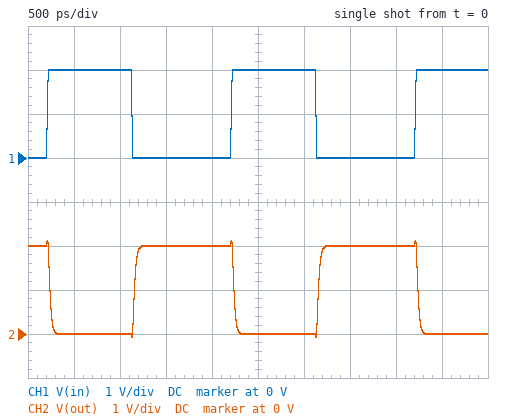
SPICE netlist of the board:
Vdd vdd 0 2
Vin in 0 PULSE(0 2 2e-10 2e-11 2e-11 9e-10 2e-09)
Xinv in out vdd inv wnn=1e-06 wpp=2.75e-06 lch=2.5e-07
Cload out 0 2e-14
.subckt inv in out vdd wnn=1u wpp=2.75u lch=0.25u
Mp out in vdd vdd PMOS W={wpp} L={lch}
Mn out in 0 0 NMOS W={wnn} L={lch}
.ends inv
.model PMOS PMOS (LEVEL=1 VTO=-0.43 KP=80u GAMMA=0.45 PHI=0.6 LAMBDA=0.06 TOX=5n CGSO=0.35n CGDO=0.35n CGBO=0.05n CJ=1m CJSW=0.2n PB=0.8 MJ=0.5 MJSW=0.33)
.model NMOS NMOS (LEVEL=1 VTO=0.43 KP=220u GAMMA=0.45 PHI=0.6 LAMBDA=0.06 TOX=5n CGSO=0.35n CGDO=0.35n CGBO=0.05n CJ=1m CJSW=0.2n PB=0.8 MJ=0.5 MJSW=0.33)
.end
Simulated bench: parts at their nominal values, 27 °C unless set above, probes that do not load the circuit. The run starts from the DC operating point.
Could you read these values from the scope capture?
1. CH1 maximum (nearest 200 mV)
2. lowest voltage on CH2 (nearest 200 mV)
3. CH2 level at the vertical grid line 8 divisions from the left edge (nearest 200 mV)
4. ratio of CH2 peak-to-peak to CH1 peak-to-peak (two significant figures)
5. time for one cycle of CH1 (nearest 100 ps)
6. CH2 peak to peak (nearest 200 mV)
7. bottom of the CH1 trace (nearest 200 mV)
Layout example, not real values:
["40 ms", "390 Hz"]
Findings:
["2.0 V", "0 V", "2.0 V", "1.1", "2.0 ns", "2.2 V", "0 V"]
